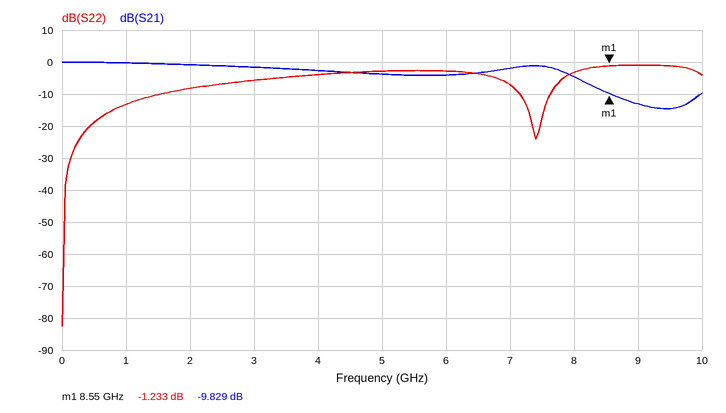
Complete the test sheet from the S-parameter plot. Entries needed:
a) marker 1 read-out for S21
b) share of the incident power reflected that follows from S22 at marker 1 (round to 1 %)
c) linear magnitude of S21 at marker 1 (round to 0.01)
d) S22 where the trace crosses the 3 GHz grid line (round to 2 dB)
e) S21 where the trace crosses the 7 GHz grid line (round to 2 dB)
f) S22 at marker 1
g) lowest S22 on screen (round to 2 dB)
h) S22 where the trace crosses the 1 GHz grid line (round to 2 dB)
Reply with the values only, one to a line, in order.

-9.829 dB
75 %
0.32
-6 dB
-2 dB
-1.233 dB
-82 dB
-14 dB
